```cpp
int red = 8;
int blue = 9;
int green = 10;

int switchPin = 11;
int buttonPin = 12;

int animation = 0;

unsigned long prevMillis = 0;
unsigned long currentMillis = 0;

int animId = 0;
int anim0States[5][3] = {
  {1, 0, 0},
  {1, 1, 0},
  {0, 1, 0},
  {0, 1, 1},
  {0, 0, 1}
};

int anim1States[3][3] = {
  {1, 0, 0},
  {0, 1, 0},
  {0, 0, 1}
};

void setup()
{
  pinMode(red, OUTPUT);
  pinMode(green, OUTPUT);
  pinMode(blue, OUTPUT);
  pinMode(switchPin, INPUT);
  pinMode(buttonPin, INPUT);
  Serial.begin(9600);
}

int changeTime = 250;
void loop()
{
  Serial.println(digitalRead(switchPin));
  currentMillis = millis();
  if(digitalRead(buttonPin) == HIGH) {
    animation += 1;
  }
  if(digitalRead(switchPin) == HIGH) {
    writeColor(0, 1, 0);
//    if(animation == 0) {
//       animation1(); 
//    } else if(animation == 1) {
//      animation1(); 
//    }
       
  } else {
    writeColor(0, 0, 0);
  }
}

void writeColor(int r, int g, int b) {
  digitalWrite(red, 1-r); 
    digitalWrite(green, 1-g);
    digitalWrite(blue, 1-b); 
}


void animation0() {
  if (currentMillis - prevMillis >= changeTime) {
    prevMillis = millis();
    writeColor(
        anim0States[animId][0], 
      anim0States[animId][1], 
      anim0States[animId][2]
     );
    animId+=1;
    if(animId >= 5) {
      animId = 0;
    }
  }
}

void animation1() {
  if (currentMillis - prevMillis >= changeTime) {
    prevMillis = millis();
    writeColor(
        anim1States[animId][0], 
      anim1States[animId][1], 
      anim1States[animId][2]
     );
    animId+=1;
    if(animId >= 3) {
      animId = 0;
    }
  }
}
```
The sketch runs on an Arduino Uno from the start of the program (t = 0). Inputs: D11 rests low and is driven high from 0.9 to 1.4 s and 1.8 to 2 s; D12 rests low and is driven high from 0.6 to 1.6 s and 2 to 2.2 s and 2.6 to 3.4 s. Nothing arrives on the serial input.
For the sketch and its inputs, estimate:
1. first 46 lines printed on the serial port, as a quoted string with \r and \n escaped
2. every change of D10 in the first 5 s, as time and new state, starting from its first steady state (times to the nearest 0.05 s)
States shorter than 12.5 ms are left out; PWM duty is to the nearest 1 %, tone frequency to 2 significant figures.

"0\r\n0\r\n0\r\n0\r\n0\r\n0\r\n0\r\n0\r\n0\r\n0\r\n0\r\n0\r\n0\r\n0\r\n0\r\n0\r\n0\r\n0\r\n0\r\n0\r\n0\r\n0\r\n0\r\n0\r\n0\r\n0\r\n0\r\n0\r\n0\r\n0\r\n0\r\n0\r\n0\r\n0\r\n0\r\n0\r\n0\r\n0\r\n0\r\n0\r\n0\r\n0\r\n0\r\n0\r\n0\r\n0\r\n"
0 s high; 0.9 s low; 1.4 s high; 1.8 s low; 2 s high
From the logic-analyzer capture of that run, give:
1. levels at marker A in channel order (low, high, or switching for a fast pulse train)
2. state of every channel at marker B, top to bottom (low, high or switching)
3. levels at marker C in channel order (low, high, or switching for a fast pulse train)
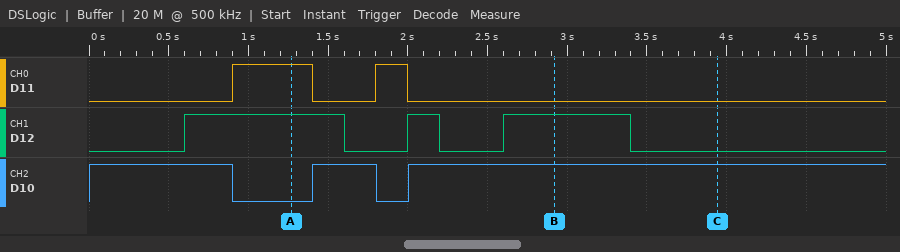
D11 high, D12 high, D10 low
D11 low, D12 high, D10 high
D11 low, D12 low, D10 high
